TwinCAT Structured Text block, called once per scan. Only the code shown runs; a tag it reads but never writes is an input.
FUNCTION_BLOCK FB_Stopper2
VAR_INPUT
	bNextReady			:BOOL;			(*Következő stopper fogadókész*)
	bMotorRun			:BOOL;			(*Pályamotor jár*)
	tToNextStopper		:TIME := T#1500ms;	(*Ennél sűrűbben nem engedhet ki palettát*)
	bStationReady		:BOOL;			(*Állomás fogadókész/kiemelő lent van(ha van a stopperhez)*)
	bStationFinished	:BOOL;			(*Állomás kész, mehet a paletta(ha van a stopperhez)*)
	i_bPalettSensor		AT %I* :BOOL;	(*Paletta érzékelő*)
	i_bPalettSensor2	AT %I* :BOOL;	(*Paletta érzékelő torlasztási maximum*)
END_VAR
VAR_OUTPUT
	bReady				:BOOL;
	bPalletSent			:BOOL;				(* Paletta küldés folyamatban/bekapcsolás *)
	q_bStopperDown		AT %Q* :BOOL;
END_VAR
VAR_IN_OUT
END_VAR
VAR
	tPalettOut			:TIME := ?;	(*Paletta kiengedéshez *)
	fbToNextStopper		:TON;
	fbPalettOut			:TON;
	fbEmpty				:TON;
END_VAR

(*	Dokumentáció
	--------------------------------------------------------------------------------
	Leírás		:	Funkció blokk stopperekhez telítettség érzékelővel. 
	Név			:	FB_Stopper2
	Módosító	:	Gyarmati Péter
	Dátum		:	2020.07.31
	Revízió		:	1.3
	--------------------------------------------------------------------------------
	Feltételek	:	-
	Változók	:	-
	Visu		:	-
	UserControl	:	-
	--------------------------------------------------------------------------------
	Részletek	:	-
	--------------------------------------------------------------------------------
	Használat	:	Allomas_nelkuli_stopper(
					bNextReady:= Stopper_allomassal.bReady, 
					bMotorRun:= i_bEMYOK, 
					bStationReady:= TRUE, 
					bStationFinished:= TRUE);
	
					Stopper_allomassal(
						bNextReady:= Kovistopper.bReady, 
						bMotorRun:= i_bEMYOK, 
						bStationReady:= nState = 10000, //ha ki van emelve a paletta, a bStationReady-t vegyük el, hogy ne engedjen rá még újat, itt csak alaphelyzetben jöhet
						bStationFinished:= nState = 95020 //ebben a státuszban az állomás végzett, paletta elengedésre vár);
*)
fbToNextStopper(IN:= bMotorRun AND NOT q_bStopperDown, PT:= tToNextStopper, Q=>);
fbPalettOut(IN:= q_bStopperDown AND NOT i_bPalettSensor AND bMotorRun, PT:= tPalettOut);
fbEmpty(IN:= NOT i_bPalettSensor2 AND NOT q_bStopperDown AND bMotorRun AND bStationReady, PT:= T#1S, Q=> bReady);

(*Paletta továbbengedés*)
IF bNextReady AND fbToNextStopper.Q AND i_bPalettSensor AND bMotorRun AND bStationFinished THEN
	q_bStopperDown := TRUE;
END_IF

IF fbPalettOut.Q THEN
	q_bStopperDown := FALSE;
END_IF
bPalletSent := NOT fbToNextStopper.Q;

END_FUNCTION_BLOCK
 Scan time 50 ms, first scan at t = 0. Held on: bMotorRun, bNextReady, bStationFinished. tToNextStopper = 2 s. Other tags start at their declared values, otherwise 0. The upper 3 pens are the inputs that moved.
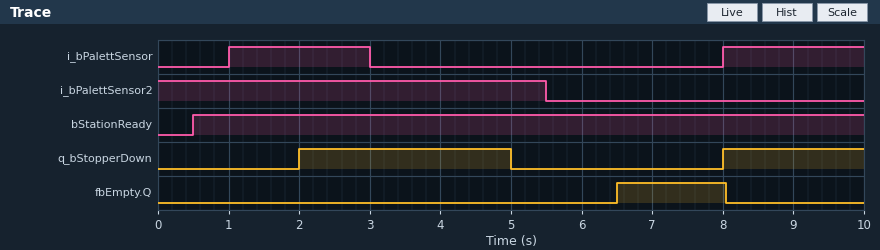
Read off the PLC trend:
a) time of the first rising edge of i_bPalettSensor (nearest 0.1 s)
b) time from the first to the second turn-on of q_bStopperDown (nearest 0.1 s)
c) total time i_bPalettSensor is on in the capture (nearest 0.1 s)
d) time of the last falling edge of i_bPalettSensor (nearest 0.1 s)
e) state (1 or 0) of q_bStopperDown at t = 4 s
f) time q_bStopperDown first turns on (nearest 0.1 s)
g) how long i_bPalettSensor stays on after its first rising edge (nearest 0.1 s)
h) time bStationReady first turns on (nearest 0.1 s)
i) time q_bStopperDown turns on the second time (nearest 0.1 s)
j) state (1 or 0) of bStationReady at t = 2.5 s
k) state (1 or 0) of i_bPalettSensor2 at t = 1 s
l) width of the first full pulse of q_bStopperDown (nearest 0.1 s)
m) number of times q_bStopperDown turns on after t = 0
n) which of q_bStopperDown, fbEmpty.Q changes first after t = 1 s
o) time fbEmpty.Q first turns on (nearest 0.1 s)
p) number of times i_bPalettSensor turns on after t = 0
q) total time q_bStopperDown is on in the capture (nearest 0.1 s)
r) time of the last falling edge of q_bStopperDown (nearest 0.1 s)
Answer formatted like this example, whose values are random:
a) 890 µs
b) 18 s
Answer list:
a) 1.0 s
b) 6.0 s
c) 4.0 s
d) 3.0 s
e) 1
f) 2.0 s
g) 2.0 s
h) 0.5 s
i) 8.0 s
j) 1
k) 1
l) 3.0 s
m) 2
n) q_bStopperDown
o) 6.5 s
p) 2
q) 5.0 s
r) 5.0 s
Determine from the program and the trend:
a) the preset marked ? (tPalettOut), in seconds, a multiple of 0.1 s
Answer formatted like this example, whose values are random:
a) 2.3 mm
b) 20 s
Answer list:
a) 2.0 s
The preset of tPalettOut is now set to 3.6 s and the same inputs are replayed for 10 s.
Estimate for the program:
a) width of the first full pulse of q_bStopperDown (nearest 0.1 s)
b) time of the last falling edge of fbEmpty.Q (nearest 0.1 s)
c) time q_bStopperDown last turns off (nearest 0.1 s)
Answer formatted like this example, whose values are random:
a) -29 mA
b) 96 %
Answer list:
a) 4.6 s
b) 8.7 s
c) 6.6 s
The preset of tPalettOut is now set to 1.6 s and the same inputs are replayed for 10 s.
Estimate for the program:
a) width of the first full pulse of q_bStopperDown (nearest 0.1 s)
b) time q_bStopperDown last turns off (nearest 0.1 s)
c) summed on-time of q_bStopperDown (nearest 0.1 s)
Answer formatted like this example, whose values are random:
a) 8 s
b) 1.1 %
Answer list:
a) 2.6 s
b) 4.6 s
c) 4.6 s
